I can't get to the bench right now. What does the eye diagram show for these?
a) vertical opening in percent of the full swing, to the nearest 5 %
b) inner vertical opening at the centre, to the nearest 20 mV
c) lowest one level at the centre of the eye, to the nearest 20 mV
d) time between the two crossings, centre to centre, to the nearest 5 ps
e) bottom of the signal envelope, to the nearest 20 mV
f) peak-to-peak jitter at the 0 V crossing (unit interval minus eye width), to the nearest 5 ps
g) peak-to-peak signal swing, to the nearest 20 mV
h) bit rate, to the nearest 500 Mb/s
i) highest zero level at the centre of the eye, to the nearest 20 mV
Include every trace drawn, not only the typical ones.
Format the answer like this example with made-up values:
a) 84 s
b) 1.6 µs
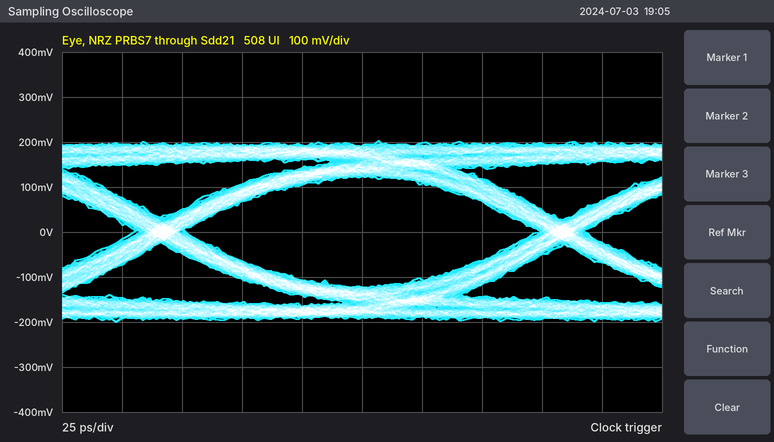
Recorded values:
a) 60 %
b) 240 mV
c) 120 mV
d) 165 ps
e) -200 mV
f) 20 ps
g) 400 mV
h) 6.0 Gb/s
i) -120 mV
